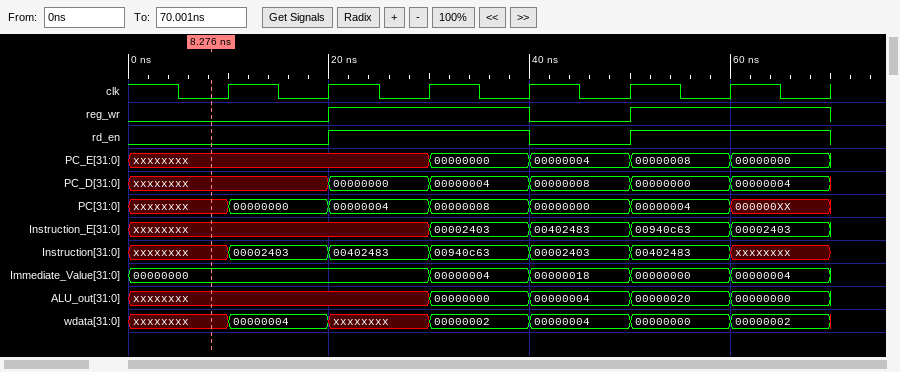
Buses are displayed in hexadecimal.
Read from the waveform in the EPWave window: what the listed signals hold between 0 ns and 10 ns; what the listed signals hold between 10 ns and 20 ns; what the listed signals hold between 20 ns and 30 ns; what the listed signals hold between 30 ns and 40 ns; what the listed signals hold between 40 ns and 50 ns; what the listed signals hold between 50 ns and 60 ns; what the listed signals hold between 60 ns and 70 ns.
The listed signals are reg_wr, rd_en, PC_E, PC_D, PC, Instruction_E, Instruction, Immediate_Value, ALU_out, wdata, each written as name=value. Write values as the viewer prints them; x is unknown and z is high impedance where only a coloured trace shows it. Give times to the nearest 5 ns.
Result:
reg_wr=0, rd_en=0, PC_E=xxxxxxxx, PC_D=xxxxxxxx, PC=xxxxxxxx, Instruction_E=xxxxxxxx, Instruction=xxxxxxxx, Immediate_Value=00000000, ALU_out=xxxxxxxx, wdata=xxxxxxxx
reg_wr=0, rd_en=0, PC_E=xxxxxxxx, PC_D=xxxxxxxx, PC=00000000, Instruction_E=xxxxxxxx, Instruction=00002403, Immediate_Value=00000000, ALU_out=xxxxxxxx, wdata=00000004
reg_wr=1, rd_en=1, PC_E=xxxxxxxx, PC_D=00000000, PC=00000004, Instruction_E=xxxxxxxx, Instruction=00402483, Immediate_Value=00000000, ALU_out=xxxxxxxx, wdata=xxxxxxxx
reg_wr=1, rd_en=1, PC_E=00000000, PC_D=00000004, PC=00000008, Instruction_E=00002403, Instruction=00940c63, Immediate_Value=00000004, ALU_out=00000000, wdata=00000002
reg_wr=0, rd_en=0, PC_E=00000004, PC_D=00000008, PC=00000000, Instruction_E=00402483, Instruction=00002403, Immediate_Value=00000018, ALU_out=00000004, wdata=00000004
reg_wr=1, rd_en=1, PC_E=00000008, PC_D=00000000, PC=00000004, Instruction_E=00940c63, Instruction=00402483, Immediate_Value=00000000, ALU_out=00000020, wdata=00000000
reg_wr=1, rd_en=1, PC_E=00000000, PC_D=00000004, PC=000000XX, Instruction_E=00002403, Instruction=xxxxxxxx, Immediate_Value=00000004, ALU_out=00000000, wdata=00000002
